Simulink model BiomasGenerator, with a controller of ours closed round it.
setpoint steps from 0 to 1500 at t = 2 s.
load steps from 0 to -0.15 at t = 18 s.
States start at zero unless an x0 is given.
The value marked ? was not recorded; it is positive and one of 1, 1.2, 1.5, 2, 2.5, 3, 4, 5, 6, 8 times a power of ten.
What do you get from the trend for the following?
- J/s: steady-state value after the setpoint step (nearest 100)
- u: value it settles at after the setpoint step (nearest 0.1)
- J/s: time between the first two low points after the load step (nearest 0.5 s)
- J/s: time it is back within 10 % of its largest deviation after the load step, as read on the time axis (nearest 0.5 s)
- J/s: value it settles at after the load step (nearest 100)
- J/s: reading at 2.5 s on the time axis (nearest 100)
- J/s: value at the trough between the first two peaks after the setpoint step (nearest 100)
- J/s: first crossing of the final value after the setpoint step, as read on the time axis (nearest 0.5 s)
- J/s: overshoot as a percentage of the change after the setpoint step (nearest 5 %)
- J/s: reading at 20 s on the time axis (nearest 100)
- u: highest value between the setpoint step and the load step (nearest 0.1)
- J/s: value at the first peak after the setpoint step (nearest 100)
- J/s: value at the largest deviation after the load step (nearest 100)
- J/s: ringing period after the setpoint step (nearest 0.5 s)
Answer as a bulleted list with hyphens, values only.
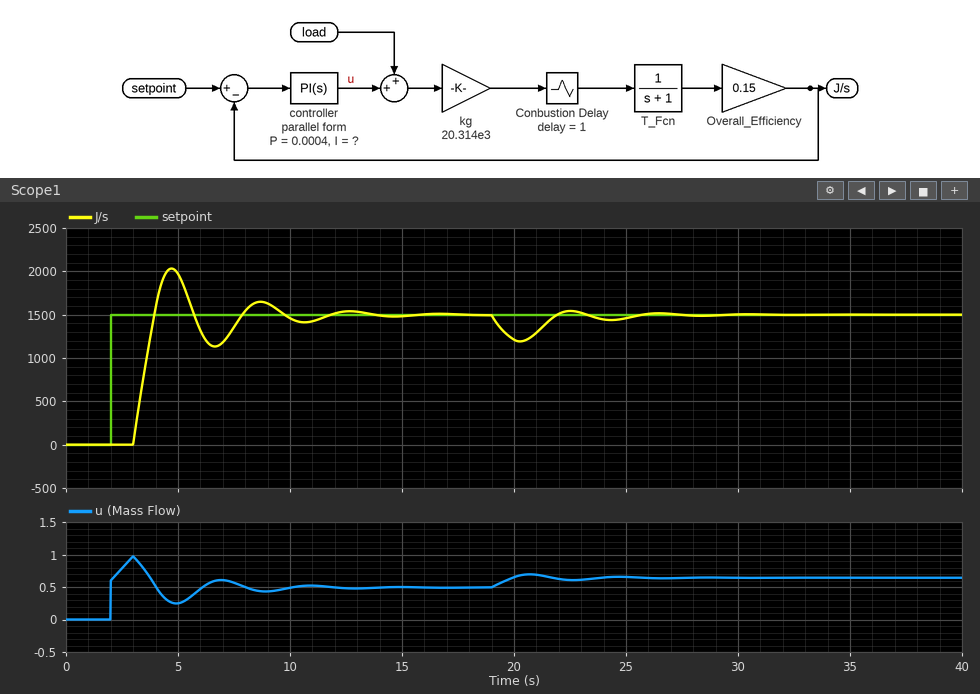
- 1500
- 0.5
- 4.0 s
- 25.0 s
- 1500
- 0
- 1100
- 4.0 s
- 35 %
- 1200
- 1.0
- 2000
- 1200
- 4.0 s
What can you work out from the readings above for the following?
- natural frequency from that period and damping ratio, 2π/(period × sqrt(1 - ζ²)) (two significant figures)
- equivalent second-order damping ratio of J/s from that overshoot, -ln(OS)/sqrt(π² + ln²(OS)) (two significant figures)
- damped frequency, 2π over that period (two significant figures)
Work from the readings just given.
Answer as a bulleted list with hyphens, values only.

- 1.7 rad/s
- 0.32
- 1.6 rad/s
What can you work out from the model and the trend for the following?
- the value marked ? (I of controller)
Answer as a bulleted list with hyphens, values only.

- 0.00025
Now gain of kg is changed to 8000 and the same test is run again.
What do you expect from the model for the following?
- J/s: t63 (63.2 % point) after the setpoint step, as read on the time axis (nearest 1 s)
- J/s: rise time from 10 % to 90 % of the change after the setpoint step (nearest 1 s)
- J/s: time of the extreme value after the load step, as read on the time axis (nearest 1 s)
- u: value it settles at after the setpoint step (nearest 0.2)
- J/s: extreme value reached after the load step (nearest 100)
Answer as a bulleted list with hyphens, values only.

- 5 s
- 6 s
- 21 s
- 1.2
- 1400
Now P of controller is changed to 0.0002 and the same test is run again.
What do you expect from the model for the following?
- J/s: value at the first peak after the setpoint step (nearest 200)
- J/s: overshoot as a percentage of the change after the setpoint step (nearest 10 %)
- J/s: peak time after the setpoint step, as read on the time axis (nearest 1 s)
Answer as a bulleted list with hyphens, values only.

- 2000
- 30 %
- 6 s
